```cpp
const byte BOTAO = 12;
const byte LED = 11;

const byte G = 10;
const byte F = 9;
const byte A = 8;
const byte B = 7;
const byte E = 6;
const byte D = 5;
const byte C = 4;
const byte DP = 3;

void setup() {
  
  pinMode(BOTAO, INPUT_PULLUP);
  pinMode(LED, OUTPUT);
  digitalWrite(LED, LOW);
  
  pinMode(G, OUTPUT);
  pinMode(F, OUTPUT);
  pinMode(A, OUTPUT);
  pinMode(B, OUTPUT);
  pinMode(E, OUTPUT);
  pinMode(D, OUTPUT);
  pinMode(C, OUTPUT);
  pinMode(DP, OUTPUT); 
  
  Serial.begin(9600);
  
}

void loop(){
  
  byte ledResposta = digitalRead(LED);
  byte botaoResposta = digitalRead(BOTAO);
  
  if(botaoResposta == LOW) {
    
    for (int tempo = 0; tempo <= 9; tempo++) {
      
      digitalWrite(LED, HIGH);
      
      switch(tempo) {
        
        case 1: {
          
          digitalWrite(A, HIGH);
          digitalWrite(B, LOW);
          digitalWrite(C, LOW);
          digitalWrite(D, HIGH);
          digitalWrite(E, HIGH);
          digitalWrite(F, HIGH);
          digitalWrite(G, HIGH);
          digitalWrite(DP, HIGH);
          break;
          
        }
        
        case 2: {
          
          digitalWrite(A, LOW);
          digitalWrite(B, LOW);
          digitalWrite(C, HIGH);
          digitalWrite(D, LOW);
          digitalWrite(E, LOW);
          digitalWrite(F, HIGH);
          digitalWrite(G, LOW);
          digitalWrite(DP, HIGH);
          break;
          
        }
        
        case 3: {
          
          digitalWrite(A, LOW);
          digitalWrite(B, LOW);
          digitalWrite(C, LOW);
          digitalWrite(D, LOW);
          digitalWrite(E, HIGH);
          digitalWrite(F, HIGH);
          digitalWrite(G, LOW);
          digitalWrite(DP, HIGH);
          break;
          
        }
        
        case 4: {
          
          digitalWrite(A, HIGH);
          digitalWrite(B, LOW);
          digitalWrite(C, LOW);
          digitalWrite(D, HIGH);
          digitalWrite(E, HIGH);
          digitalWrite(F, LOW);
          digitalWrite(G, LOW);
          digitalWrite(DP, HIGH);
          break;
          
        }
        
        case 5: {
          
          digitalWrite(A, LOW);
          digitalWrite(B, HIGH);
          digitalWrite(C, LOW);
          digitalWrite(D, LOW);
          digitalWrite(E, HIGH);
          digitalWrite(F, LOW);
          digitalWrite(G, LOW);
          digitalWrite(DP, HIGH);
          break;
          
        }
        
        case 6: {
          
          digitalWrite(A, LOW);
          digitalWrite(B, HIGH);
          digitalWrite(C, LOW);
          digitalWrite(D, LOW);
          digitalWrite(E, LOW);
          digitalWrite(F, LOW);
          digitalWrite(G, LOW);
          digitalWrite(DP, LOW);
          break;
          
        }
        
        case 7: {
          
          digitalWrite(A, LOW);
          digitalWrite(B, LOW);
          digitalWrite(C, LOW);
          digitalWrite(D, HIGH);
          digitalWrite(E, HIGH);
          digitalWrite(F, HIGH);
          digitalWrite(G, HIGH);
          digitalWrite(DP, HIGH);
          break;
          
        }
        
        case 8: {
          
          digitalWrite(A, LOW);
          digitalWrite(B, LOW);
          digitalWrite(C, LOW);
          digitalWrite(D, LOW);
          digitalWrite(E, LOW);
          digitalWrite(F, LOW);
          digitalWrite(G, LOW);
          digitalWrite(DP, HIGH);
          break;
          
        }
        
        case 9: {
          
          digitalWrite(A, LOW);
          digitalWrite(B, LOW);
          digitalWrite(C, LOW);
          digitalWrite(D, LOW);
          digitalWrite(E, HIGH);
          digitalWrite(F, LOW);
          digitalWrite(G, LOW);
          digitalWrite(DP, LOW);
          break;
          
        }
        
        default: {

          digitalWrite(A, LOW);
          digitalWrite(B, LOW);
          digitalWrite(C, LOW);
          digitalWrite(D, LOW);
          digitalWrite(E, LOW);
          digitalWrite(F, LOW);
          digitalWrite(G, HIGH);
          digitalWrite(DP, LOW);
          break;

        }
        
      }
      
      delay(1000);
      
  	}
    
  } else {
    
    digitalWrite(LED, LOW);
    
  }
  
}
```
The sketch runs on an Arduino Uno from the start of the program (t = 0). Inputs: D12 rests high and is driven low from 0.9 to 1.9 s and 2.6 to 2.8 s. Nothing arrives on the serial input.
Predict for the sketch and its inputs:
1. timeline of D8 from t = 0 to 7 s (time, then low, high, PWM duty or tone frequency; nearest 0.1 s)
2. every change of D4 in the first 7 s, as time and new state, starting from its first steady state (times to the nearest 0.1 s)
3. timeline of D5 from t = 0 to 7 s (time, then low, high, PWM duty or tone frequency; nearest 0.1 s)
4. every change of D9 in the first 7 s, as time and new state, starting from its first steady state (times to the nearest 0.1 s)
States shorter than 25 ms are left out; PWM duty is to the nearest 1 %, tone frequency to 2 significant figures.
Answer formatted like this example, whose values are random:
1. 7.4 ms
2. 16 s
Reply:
1. 0 s low; 1.9 s high; 2.9 s low; 4.9 s high; 5.9 s low
2. 0 s low; 2.9 s high; 3.9 s low
3. 0 s low; 1.9 s high; 2.9 s low; 4.9 s high; 5.9 s low
4. 0 s low; 1.9 s high; 4.9 s low
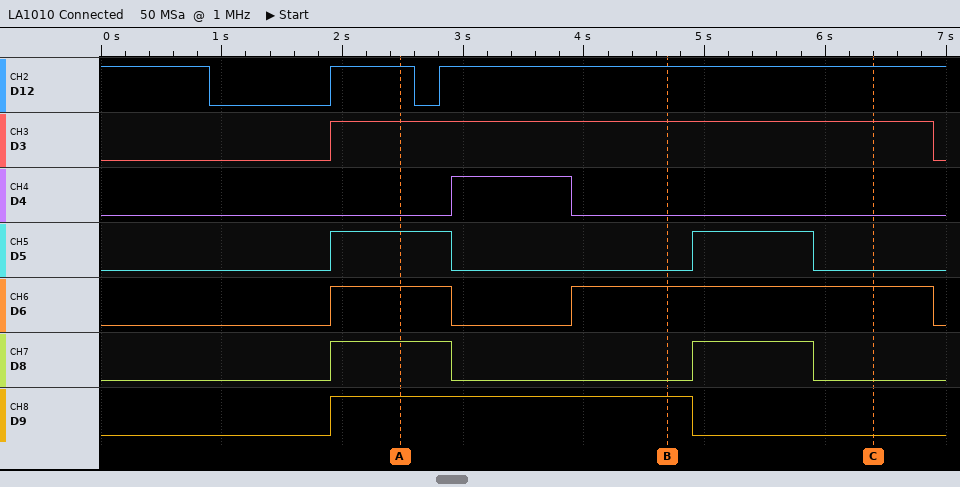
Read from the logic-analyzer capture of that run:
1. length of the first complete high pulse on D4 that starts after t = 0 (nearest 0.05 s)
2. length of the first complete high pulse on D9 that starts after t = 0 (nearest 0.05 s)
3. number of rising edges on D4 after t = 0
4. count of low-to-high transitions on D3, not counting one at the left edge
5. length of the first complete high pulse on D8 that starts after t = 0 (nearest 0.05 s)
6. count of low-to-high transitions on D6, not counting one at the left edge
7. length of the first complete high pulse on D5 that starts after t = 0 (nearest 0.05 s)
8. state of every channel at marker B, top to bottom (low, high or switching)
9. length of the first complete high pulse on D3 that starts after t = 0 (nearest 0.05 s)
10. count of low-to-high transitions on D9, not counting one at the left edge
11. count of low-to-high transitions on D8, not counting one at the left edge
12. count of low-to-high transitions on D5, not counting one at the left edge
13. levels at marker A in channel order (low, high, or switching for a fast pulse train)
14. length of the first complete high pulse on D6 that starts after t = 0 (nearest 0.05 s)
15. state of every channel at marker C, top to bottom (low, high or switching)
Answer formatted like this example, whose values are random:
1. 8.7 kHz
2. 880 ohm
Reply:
1. 1.00 s
2. 3.00 s
3. 1
4. 1
5. 1.00 s
6. 2
7. 1.00 s
8. D12 high, D3 high, D4 low, D5 low, D6 high, D8 low, D9 high
9. 5.00 s
10. 1
11. 2
12. 2
13. D12 high, D3 high, D4 low, D5 high, D6 high, D8 high, D9 high
14. 1.00 s
15. D12 high, D3 high, D4 low, D5 low, D6 high, D8 low, D9 low
